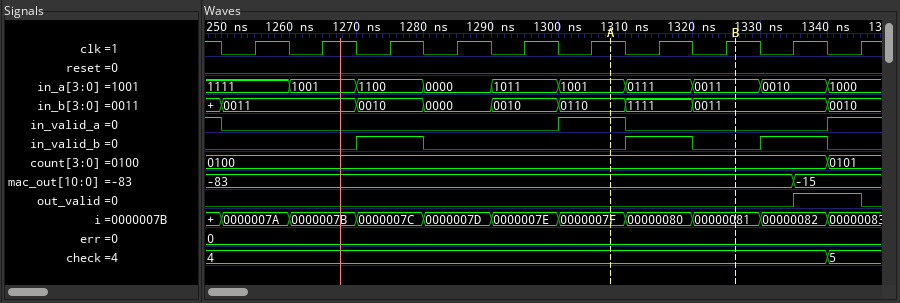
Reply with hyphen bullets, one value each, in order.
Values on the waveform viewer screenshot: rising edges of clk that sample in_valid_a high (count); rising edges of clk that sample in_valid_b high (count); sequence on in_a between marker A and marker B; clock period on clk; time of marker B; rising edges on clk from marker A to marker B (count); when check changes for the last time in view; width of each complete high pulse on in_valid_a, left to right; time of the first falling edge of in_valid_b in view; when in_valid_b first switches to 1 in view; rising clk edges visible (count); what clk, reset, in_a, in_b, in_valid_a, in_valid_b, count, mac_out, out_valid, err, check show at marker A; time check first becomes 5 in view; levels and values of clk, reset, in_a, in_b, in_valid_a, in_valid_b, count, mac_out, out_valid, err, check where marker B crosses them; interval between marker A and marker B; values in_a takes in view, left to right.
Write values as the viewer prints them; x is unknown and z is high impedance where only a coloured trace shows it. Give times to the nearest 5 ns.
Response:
- 2
- 3
- 1001, 0111, 0011
- 10 ns
- 1325 ns
- 2
- 1340 ns
- 10 ns
- 1280 ns
- 1270 ns
- 10
- clk=1, reset=0, in_a=1001, in_b=0110, in_valid_a=1, in_valid_b=0, count=0100, mac_out=-83, out_valid=0, err=0, check=4
- 1340 ns
- clk=1, reset=0, in_a=0011, in_b=0011, in_valid_a=0, in_valid_b=0, count=0100, mac_out=-83, out_valid=0, err=0, check=4
- 20 ns
- 1111, 1001, 1100, 0000, 1011, 1001, 0111, 0011, 0010, 1000
